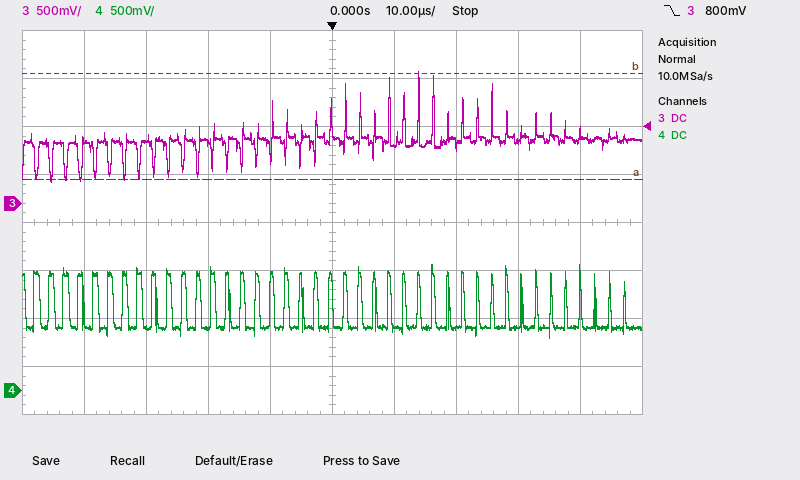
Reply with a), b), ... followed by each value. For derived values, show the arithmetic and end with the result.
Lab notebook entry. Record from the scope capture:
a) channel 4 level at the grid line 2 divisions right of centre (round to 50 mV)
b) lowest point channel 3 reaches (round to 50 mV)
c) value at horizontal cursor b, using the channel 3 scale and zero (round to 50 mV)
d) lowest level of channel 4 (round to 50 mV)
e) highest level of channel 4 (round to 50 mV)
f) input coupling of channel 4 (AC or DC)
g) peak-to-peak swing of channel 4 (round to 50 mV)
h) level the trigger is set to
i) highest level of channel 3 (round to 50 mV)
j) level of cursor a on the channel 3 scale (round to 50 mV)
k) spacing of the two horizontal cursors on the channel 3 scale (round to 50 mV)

a) 650 mV
b) 250 mV
c) 1.35 V
d) 550 mV
e) 1.30 V
f) DC
g) 1.30 V − (550 mV) = 750 mV
h) 800 mV
i) 1.35 V
j) 250 mV
k) 1.10 V
